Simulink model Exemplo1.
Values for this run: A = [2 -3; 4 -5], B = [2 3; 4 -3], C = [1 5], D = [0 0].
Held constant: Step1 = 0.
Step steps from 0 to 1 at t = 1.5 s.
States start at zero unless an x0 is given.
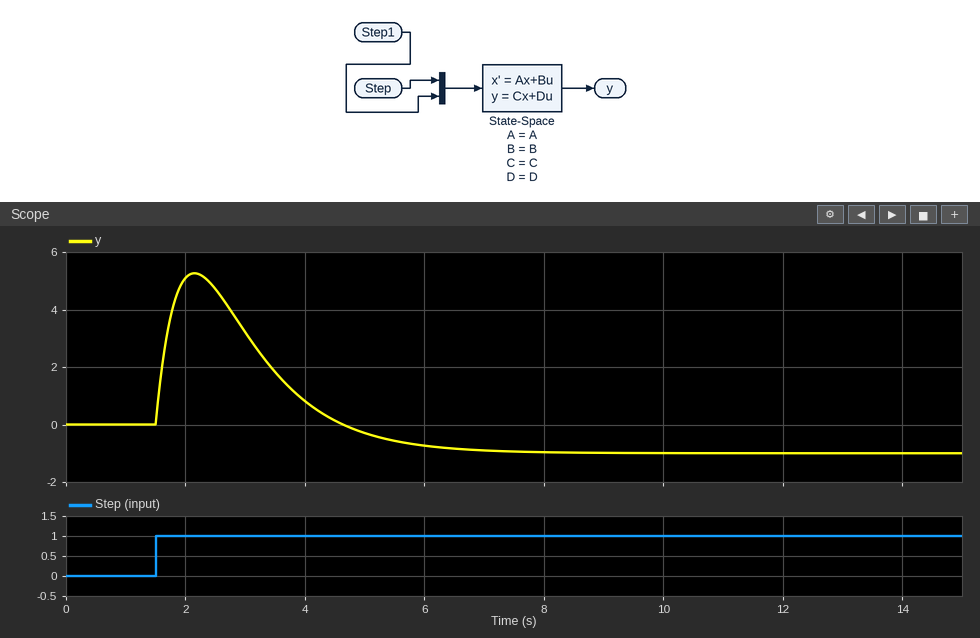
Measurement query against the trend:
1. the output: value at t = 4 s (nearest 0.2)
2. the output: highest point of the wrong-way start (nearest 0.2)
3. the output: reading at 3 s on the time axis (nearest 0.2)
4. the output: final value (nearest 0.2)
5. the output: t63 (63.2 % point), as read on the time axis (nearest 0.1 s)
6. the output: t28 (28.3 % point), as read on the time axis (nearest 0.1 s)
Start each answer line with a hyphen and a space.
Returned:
- 0.8
- 5.2
- 3.2
- -1.0
- 5.7 s
- 5.0 s
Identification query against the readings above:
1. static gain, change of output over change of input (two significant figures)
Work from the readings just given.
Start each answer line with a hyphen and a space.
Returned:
- -1.0
